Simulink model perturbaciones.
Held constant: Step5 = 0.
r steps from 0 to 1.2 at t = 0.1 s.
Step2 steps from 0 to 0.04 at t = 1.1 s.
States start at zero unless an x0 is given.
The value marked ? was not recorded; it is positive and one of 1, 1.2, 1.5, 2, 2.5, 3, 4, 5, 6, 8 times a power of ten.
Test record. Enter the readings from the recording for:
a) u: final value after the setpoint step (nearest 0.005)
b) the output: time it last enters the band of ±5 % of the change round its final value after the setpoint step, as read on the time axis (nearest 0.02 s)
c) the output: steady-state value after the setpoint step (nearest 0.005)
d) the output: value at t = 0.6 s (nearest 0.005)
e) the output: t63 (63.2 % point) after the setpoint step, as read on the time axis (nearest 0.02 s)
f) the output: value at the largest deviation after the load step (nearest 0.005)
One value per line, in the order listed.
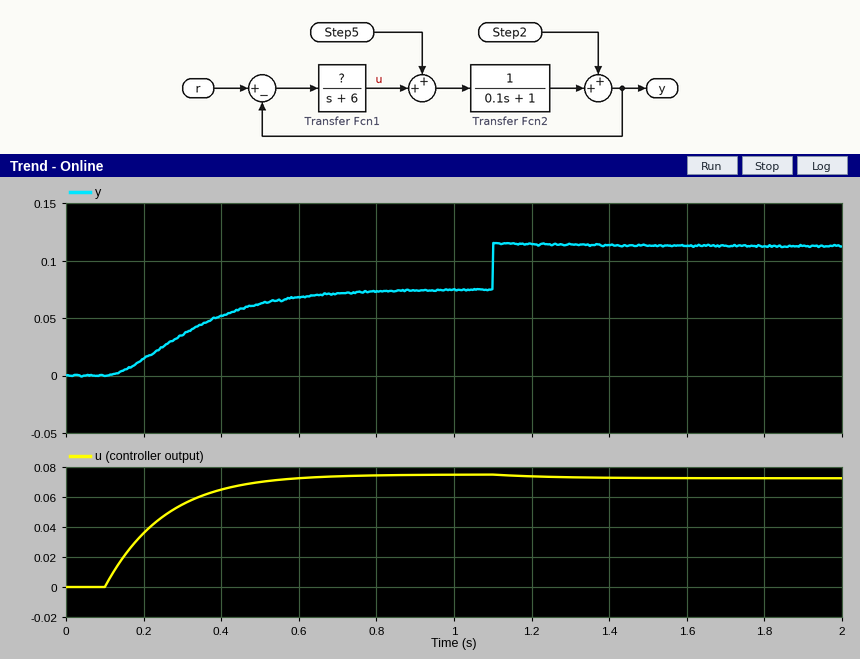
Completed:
0.075
0.70 s
0.075
0.070
0.36 s
0.115
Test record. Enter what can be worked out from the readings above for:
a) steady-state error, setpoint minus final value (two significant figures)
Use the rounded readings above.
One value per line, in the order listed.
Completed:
1.1
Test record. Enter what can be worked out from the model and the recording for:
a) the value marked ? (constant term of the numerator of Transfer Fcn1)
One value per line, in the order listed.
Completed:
0.4
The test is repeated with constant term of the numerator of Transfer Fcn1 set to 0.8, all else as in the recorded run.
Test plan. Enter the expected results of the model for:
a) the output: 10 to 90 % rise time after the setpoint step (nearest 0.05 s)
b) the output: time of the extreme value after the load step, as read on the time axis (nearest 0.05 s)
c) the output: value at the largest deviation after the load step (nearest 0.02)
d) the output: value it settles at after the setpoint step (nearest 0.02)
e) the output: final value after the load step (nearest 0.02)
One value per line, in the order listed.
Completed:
0.40 s
1.10 s
0.18
0.14
0.18
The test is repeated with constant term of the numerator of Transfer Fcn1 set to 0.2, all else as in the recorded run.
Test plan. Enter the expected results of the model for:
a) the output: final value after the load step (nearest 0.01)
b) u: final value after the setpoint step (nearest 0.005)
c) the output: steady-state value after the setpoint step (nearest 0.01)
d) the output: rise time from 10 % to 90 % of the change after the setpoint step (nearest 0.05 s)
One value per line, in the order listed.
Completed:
0.08
0.040
0.04
0.45 s
